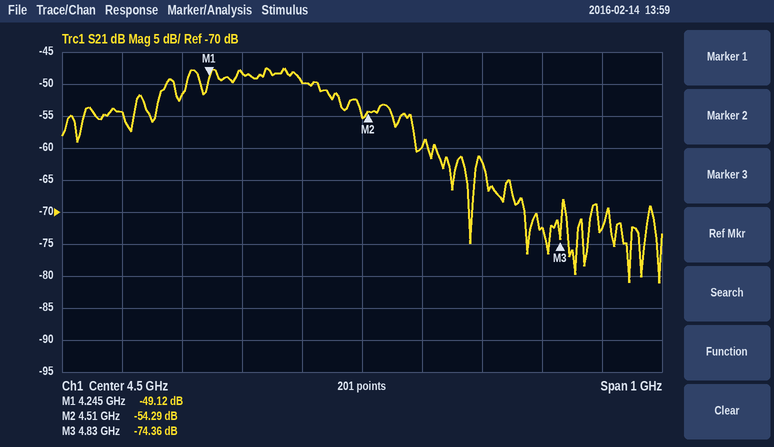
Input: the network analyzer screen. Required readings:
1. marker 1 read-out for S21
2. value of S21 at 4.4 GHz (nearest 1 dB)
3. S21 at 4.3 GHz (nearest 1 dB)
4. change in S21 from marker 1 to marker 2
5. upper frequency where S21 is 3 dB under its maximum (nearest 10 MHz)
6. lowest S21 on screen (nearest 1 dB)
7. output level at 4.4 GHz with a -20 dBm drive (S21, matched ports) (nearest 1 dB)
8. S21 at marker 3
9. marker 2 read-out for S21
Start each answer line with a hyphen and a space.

- -49.12 dB
- -50 dB
- -48 dB
- -5.17 dB
- 4.43 GHz
- -81 dB
- -70 dBm
- -74.36 dB
- -54.29 dB
